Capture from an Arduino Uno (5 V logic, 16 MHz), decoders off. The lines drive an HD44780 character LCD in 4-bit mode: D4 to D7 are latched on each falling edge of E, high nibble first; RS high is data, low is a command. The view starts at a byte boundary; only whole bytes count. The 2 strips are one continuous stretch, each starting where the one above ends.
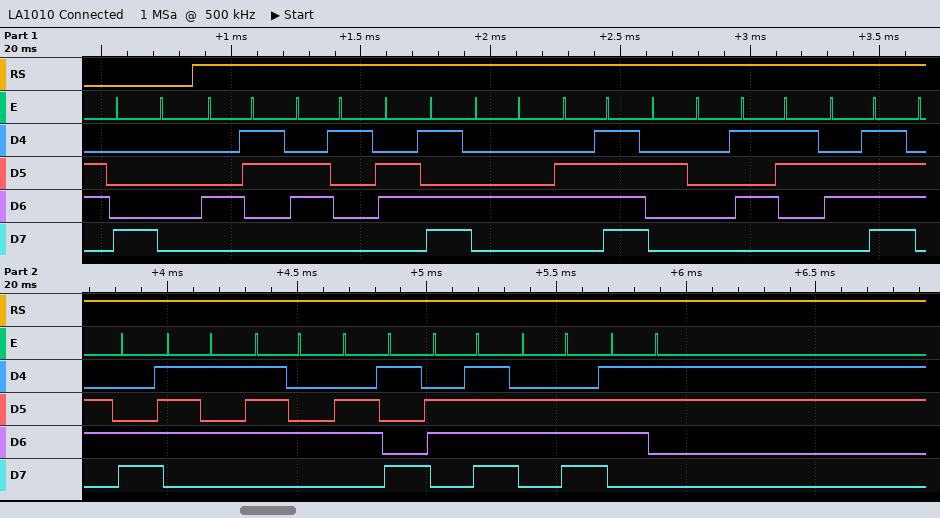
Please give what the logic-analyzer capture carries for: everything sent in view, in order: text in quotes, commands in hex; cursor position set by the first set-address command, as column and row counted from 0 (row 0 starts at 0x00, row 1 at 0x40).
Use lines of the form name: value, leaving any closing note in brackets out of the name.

everything sent in view, in order: text in quotes, commands in hex: 0x80 "CamDo Solutions"
cursor position set by the first set-address command, as column and row counted from 0: column 0, row 0
